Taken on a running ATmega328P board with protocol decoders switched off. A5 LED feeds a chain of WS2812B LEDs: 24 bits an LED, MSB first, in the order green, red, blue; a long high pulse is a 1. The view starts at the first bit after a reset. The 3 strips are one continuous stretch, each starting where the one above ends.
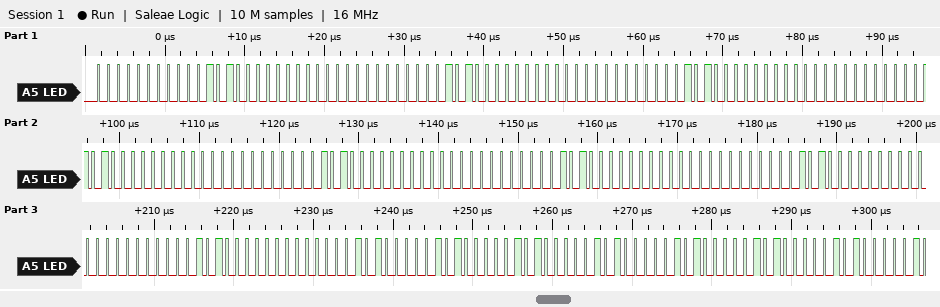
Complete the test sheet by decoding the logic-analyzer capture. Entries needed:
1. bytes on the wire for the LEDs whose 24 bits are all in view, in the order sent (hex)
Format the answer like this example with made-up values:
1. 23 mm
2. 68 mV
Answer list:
1. 00 14 00 00 14 00 00 14 00 00 14 00 00 14 00 00 14 00 00 14 00 00 14 00 14 14 14 14 14 14
